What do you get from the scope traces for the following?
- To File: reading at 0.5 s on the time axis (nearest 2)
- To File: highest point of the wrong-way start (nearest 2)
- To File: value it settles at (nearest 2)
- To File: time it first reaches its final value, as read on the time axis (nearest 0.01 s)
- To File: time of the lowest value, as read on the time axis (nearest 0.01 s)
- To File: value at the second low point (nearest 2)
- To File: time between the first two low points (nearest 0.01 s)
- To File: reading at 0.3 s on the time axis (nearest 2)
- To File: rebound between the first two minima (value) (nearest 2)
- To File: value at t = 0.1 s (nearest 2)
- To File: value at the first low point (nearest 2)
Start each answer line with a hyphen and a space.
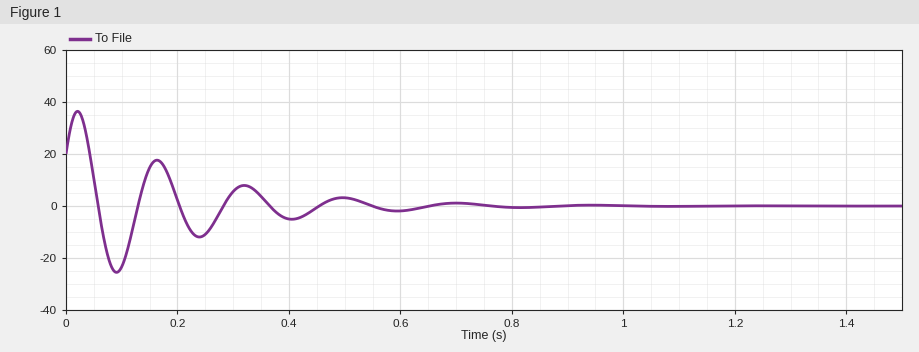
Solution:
- 4
- 36
- 0
- 0.06 s
- 0.09 s
- -12
- 0.15 s
- 6
- 18
- -24
- -26
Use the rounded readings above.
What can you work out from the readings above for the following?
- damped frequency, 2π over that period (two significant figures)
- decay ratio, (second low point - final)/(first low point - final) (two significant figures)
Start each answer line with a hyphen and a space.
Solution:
- 42 rad/s
- 0.46
